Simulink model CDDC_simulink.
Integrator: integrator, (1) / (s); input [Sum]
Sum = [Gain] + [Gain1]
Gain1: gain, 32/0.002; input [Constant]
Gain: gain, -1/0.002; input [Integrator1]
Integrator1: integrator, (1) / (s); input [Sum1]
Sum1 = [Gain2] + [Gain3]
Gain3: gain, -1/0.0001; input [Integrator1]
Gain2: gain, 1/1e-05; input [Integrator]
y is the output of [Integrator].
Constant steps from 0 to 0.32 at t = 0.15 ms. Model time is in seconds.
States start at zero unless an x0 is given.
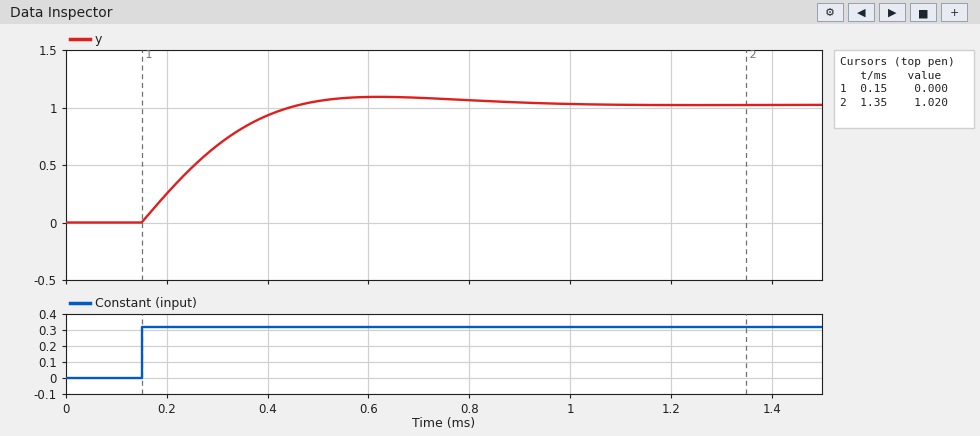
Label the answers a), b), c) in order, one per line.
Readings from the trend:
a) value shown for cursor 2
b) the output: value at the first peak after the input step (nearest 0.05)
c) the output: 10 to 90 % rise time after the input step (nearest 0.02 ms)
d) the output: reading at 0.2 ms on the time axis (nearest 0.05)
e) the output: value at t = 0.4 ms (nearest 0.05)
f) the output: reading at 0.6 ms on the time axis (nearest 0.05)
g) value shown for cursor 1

a) 1.020
b) 1.10
c) 0.22 ms
d) 0.25
e) 0.95
f) 1.10
g) 0.000
